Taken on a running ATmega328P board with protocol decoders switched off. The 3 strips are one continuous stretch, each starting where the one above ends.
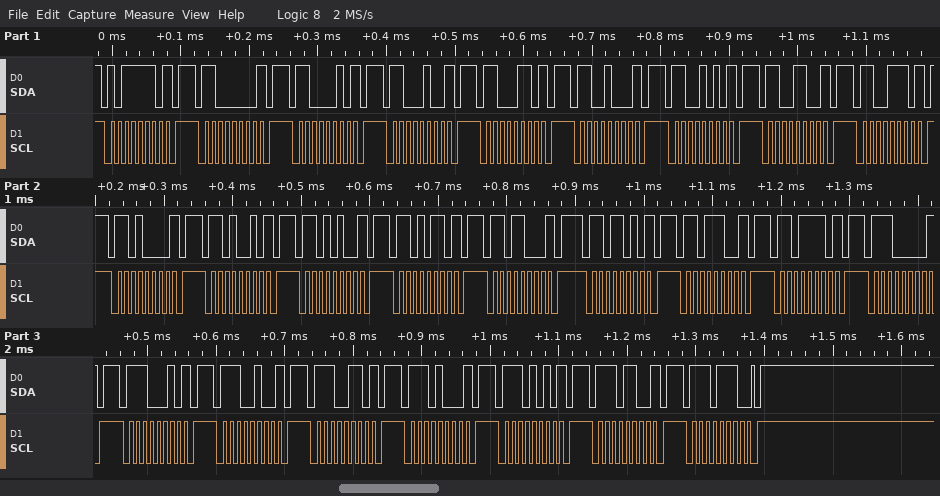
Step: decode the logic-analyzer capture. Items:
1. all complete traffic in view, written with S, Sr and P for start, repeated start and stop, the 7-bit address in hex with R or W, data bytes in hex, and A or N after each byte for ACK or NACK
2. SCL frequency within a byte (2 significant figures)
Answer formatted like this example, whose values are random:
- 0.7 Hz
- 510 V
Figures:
- S 5FW N P S 60W N P S 61W N P S 62W N P S 63W N P S 64W N P S 65W N P S 66W N P S 67W N P S 68W N P S 69W N P S 6AW N P S 6BW N P S 6CW N P S 6DW N P S 6EW N P S 6FW N P S 70W N P S 71W N P S 72W N P S 73W N P S 74W N P S 75W N P S 76W N P S 77W A P
- 100 kHz
